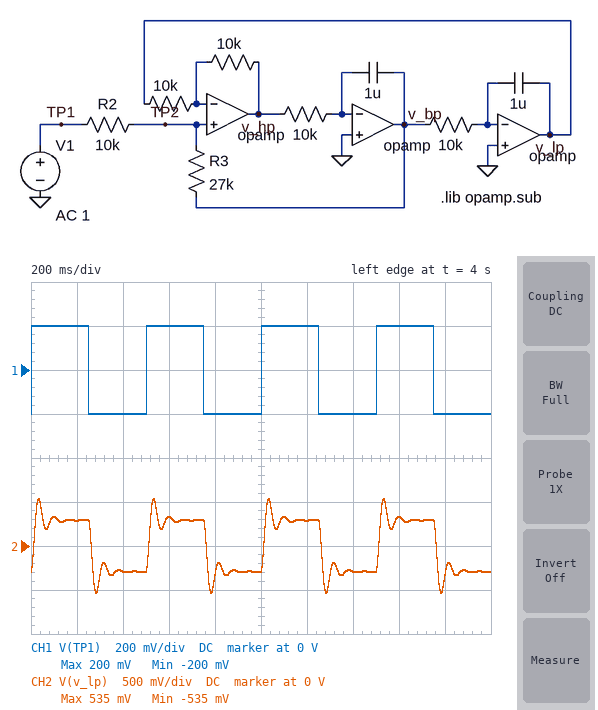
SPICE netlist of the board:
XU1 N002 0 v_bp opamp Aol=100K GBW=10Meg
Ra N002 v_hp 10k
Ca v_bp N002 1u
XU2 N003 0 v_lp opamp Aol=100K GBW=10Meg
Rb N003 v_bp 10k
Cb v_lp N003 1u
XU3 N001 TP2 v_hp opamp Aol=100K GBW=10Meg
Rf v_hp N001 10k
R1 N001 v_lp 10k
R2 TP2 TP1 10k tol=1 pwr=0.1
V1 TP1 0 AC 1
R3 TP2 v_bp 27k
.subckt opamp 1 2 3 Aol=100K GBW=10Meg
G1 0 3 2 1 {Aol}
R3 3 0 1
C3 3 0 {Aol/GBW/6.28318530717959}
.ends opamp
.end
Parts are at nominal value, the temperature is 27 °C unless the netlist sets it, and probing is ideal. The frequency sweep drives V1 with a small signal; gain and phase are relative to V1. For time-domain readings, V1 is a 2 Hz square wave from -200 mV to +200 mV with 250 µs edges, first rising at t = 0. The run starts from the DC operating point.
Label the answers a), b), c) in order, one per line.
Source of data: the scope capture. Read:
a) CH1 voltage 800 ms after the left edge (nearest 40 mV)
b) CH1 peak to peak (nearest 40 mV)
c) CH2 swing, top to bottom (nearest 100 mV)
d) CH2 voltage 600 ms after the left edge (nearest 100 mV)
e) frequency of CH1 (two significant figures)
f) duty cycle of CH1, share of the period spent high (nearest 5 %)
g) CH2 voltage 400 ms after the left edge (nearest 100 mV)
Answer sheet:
a) -200 mV
b) 400 mV
c) 1.1 V
d) 300 mV
e) 2.0 Hz
f) 50 %
g) -300 mV
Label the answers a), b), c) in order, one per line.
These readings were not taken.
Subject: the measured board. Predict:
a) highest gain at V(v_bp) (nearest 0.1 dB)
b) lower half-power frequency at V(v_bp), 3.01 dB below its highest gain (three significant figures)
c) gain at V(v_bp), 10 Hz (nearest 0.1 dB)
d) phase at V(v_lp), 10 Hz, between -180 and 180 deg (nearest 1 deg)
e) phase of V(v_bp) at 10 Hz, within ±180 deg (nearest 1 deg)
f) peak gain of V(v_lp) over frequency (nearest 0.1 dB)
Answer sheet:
a) 8.6 dB
b) 12.2 Hz
c) 2.4 dB
d) -29 deg
e) -119 deg
f) 9.0 dB
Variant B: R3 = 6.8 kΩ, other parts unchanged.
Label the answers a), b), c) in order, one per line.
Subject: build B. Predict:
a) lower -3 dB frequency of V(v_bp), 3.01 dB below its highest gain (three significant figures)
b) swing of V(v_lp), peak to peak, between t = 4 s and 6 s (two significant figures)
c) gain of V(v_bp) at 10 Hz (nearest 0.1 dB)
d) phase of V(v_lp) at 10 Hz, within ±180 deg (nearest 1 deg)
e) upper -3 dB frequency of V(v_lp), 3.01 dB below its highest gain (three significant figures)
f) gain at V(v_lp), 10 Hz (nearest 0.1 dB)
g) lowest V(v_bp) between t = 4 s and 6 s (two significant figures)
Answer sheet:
a) 9.05 Hz
b) 390 mV
c) -5.5 dB
d) -51 deg
e) 17.8 Hz
f) -1.5 dB
g) -160 mV
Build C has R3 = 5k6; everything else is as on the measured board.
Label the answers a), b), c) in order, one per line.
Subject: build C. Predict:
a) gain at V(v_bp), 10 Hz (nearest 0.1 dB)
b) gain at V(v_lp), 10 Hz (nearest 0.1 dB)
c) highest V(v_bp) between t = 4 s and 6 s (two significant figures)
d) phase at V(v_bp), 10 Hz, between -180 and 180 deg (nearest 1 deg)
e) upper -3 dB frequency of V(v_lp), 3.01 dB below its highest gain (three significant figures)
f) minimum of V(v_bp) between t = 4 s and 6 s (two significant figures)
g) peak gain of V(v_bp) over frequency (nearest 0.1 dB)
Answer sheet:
a) -7.0 dB
b) -2.9 dB
c) 140 mV
d) -143 deg
e) 17.2 Hz
f) -140 mV
g) -5.0 dB
